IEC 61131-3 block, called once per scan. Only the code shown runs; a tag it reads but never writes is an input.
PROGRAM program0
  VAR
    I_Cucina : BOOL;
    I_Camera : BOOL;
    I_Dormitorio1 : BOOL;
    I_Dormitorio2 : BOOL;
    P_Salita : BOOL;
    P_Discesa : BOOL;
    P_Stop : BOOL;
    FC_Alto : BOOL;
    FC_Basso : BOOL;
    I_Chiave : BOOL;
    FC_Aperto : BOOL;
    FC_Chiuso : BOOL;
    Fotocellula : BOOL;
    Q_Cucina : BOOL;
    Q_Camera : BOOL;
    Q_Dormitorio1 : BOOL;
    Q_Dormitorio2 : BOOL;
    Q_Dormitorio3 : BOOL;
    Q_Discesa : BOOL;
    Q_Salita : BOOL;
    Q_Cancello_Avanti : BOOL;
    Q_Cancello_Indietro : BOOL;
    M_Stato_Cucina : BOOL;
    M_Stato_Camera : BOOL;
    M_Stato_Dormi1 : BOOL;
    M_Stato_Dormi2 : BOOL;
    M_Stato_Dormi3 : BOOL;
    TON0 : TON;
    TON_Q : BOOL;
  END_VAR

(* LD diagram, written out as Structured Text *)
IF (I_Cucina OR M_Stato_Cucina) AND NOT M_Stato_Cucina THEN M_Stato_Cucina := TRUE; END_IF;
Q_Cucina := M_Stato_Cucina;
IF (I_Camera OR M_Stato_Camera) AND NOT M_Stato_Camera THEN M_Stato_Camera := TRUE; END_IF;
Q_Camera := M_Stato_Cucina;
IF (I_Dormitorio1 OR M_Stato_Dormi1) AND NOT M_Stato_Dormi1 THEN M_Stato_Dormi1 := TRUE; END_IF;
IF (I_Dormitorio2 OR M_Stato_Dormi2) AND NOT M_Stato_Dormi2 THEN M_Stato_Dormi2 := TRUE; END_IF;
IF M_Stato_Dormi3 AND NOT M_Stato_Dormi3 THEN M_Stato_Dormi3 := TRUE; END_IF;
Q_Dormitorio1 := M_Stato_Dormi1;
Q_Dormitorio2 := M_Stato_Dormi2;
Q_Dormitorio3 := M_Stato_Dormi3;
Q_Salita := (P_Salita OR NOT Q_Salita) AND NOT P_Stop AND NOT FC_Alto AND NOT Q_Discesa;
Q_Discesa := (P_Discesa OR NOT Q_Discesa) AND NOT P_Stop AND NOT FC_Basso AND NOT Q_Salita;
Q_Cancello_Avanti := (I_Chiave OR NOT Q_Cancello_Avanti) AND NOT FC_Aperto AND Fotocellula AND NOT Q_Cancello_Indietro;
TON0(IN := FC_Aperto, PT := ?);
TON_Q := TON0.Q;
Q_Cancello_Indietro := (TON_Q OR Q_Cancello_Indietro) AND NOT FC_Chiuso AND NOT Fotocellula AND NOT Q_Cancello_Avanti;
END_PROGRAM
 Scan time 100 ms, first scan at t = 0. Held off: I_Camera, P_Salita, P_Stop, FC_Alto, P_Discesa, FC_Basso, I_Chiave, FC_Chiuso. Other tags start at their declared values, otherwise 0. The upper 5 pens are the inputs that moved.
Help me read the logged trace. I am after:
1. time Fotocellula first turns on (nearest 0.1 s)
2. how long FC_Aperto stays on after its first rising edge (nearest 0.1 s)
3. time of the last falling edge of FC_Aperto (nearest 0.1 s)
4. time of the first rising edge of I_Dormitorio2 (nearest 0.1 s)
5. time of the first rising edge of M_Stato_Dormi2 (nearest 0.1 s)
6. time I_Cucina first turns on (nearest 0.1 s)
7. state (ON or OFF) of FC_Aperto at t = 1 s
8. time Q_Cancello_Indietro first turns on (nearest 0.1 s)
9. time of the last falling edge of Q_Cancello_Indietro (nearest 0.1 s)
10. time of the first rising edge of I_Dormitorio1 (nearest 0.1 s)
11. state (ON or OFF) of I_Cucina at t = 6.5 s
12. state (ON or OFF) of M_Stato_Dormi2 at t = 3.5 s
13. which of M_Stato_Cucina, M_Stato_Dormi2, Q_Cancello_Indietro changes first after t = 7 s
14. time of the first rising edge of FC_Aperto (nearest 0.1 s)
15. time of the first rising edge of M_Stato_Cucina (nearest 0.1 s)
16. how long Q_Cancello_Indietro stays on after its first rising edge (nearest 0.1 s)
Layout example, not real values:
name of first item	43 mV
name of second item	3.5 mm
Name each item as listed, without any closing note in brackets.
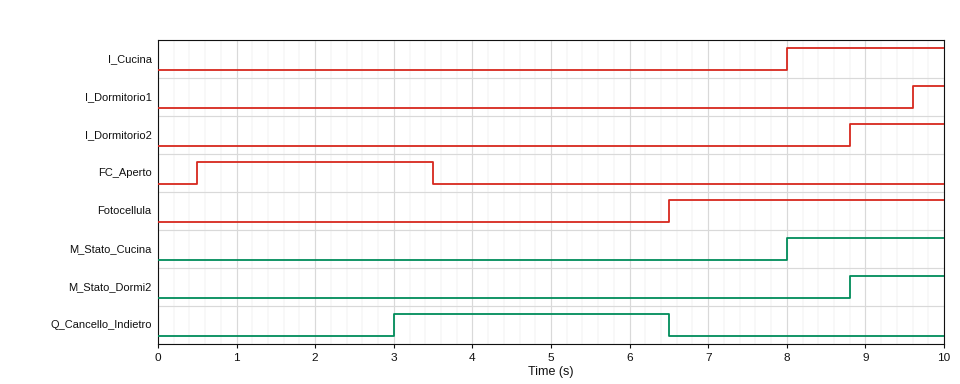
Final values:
time Fotocellula first turns on	6.5 s
how long FC_Aperto stays on after its first rising edge	3.0 s
time of the last falling edge of FC_Aperto	3.5 s
time of the first rising edge of I_Dormitorio2	8.8 s
time of the first rising edge of M_Stato_Dormi2	8.8 s
time I_Cucina first turns on	8.0 s
state (ON or OFF) of FC_Aperto at t = 1 s	ON
time Q_Cancello_Indietro first turns on	3.0 s
time of the last falling edge of Q_Cancello_Indietro	6.5 s
time of the first rising edge of I_Dormitorio1	9.6 s
state (ON or OFF) of I_Cucina at t = 6.5 s	OFF
state (ON or OFF) of M_Stato_Dormi2 at t = 3.5 s	OFF
which of M_Stato_Cucina, M_Stato_Dormi2, Q_Cancello_Indietro changes first after t = 7 s	M_Stato_Cucina
time of the first rising edge of FC_Aperto	0.5 s
time of the first rising edge of M_Stato_Cucina	8.0 s
how long Q_Cancello_Indietro stays on after its first rising edge	3.5 s
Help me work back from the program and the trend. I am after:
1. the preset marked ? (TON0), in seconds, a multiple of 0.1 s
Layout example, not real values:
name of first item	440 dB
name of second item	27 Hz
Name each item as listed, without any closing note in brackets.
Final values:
the preset marked ? (TON0), in seconds, a multiple of 0.1 s	2.5 s
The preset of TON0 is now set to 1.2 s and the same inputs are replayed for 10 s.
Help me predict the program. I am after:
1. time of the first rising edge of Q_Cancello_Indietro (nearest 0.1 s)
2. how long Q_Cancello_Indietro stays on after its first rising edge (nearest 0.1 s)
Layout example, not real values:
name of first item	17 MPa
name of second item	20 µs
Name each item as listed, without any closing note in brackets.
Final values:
time of the first rising edge of Q_Cancello_Indietro	1.7 s
how long Q_Cancello_Indietro stays on after its first rising edge	4.8 s
